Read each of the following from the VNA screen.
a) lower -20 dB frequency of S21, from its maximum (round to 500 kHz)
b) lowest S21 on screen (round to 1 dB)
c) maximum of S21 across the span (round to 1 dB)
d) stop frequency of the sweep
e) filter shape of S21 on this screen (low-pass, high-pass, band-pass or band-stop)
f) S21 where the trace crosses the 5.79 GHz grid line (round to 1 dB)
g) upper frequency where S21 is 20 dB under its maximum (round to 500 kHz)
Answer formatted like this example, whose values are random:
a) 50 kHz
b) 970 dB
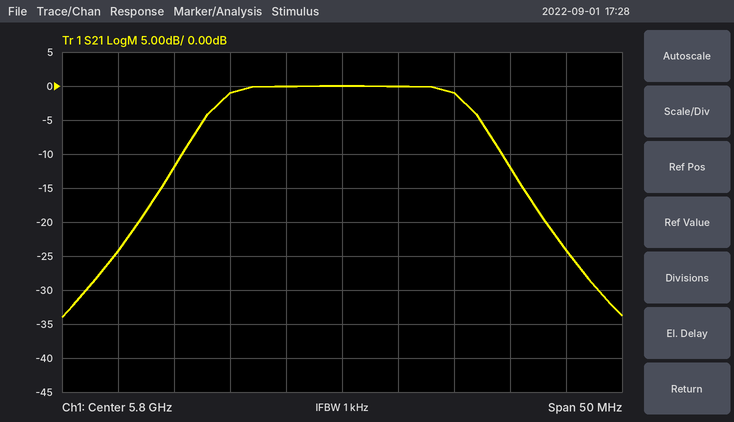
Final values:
a) 5.7820 GHz
b) -34 dB
c) 0 dB
d) 5.825 GHz
e) band-pass
f) -1 dB
g) 5.8180 GHz
